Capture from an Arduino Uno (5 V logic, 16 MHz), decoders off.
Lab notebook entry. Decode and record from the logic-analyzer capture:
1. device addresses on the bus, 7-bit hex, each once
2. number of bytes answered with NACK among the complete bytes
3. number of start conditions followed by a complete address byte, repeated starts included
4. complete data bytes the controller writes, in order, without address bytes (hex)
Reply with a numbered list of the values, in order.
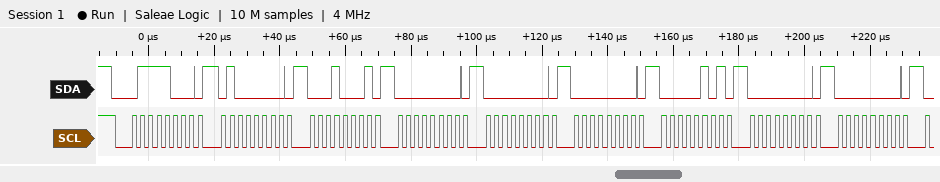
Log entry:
1. 0x3C
2. 0
3. 1
4. 40 11 00 00 00 05 00 00
